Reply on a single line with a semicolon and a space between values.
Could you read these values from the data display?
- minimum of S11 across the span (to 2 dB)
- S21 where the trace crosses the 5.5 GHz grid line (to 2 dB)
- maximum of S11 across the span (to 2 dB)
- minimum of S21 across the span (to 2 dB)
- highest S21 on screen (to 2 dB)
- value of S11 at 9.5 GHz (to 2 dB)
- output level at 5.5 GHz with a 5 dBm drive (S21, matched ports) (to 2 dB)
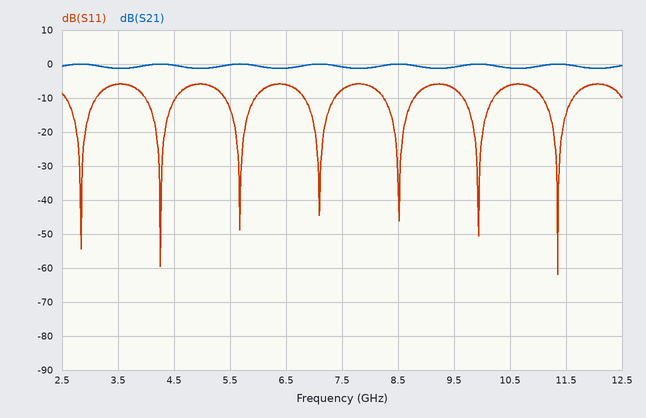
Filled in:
-62 dB; 0 dB; -6 dB; -2 dB; 0 dB; -8 dB; 4 dBm
